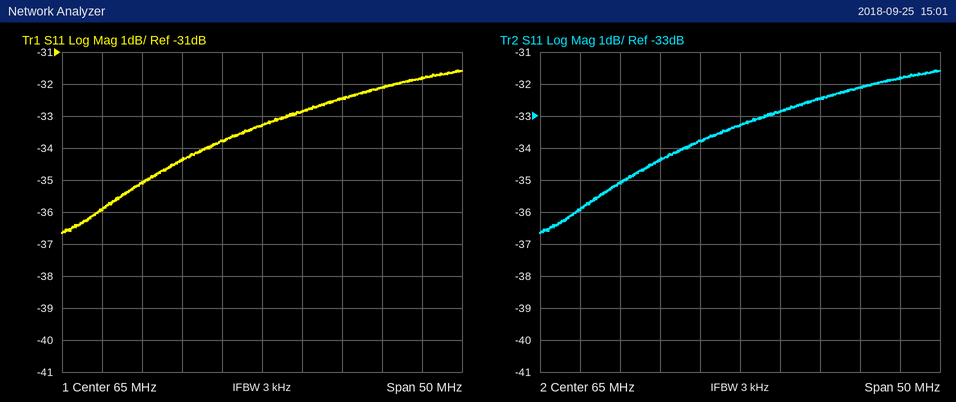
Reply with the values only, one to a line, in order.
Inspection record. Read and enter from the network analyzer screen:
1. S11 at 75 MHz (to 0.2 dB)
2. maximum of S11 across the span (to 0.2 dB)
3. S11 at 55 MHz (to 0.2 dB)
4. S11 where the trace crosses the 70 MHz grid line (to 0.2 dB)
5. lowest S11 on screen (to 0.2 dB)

-32.4 dB
-31.6 dB
-34.4 dB
-32.8 dB
-36.6 dB
